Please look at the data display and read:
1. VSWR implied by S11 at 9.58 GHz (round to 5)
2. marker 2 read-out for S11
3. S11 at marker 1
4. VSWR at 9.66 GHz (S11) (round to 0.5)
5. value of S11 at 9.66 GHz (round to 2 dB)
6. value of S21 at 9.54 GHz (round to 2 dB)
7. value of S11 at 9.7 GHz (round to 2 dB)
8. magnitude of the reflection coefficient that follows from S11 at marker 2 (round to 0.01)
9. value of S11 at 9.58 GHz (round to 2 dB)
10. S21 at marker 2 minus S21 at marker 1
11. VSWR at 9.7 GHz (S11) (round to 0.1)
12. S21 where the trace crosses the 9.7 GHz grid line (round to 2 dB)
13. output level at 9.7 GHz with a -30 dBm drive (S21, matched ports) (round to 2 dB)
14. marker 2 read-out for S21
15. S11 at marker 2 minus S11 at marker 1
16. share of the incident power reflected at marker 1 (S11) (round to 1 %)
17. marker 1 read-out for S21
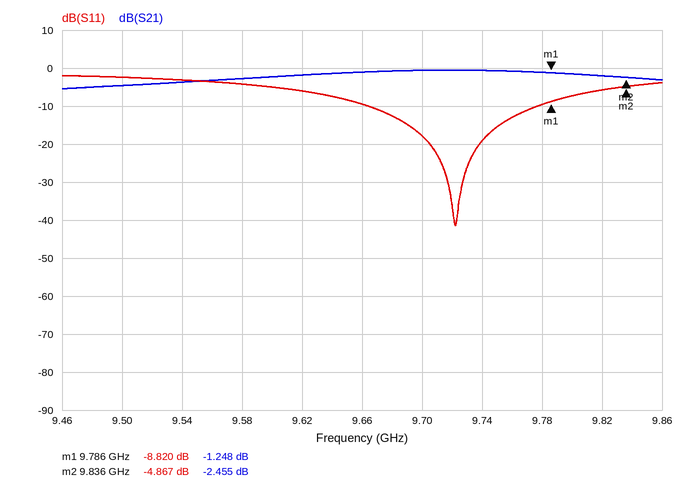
5
-4.867 dB
-8.820 dB
2.0
-10 dB
-4 dB
-18 dB
0.57
-4 dB
-1.207 dB
1.3
0 dB
-30 dBm
-2.455 dB
3.953 dB
13 %
-1.248 dB
